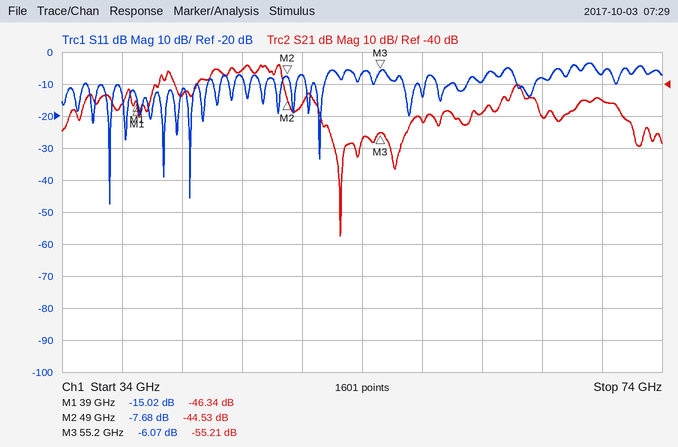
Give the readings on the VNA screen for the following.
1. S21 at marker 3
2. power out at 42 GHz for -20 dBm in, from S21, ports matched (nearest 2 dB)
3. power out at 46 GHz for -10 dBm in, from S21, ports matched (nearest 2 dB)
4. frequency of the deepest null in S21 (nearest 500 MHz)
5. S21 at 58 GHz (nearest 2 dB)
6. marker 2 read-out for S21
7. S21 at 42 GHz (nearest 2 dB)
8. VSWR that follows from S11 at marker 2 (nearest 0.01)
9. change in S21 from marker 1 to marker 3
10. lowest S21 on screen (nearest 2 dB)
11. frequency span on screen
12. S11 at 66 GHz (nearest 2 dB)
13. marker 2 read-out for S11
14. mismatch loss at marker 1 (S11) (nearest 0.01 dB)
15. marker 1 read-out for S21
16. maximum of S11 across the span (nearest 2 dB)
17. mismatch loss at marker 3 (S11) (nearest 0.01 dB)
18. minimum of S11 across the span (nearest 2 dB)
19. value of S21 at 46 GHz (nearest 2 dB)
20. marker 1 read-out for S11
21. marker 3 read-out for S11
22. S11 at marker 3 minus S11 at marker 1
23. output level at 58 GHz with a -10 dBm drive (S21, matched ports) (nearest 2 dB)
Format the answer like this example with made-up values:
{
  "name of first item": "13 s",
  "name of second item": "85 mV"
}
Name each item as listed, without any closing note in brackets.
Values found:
{
  "S21 at marker 3": "-55.21 dB",
  "power out at 42 GHz for -20 dBm in, from S21, ports matched": "-64 dBm",
  "power out at 46 GHz for -10 dBm in, from S21, ports matched": "-46 dBm",
  "frequency of the deepest null in S21": "52.5 GHz",
  "S21 at 58 GHz": "-52 dB",
  "marker 2 read-out for S21": "-44.53 dB",
  "S21 at 42 GHz": "-44 dB",
  "VSWR that follows from S11 at marker 2": "2.41",
  "change in S21 from marker 1 to marker 3": "-8.87 dB",
  "lowest S21 on screen": "-88 dB",
  "frequency span on screen": "40 GHz",
  "S11 at 66 GHz": "-8 dB",
  "marker 2 read-out for S11": "-7.68 dB",
  "mismatch loss at marker 1 (S11)": "0.14 dB",
  "marker 1 read-out for S21": "-46.34 dB",
  "maximum of S11 across the span": "-4 dB",
  "mismatch loss at marker 3 (S11)": "1.23 dB",
  "minimum of S11 across the span": "-48 dB",
  "value of S21 at 46 GHz": "-36 dB",
  "marker 1 read-out for S11": "-15.02 dB",
  "marker 3 read-out for S11": "-6.07 dB",
  "S11 at marker 3 minus S11 at marker 1": "8.95 dB",
  "output level at 58 GHz with a -10 dBm drive (S21, matched ports)": "-62 dBm"
}
